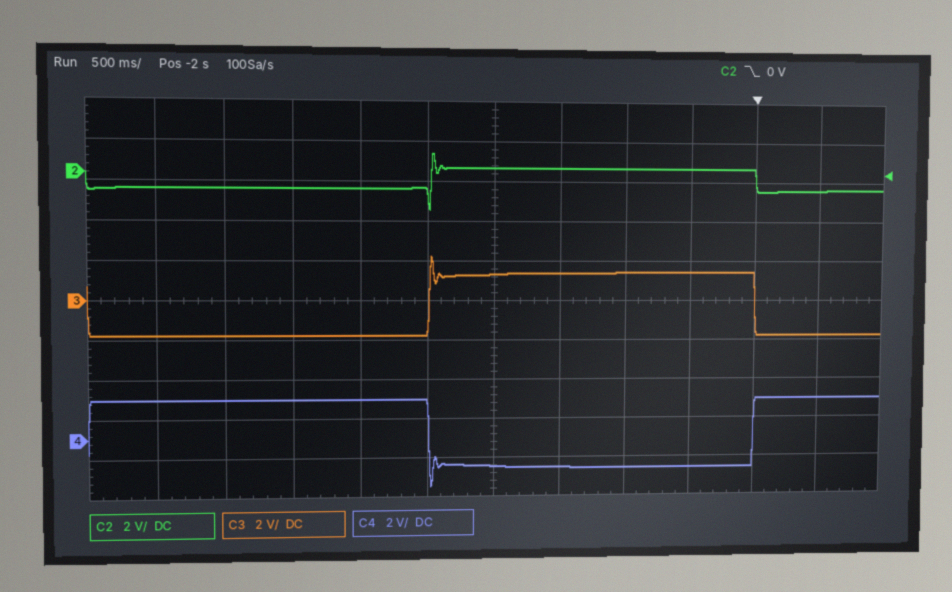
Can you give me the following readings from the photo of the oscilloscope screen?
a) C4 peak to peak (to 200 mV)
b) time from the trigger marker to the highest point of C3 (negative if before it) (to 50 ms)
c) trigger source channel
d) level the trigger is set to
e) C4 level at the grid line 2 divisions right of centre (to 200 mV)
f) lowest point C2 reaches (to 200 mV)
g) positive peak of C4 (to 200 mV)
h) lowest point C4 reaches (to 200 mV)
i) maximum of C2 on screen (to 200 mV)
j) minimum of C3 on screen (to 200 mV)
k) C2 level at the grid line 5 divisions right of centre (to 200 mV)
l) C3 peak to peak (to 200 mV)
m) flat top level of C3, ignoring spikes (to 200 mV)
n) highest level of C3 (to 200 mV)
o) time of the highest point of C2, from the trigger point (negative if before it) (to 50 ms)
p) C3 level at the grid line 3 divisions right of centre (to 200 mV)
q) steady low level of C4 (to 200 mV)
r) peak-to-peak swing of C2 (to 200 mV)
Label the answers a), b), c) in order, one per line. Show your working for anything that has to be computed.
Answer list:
a) 2.0 V − (-2.4 V) = 4.4 V
b) -2.45 s
c) C2
d) 0 V
e) -1.6 V
f) -1.8 V
g) 2.0 V
h) -2.4 V
i) 1.0 V
j) -1.8 V
k) -800 mV
l) 2.2 V − (-1.8 V) = 4.0 V
m) 1.4 V
n) 2.2 V
o) -2.45 s
p) 1.4 V
q) -1.6 V
r) 1.0 V − (-1.8 V) = 2.8 V
